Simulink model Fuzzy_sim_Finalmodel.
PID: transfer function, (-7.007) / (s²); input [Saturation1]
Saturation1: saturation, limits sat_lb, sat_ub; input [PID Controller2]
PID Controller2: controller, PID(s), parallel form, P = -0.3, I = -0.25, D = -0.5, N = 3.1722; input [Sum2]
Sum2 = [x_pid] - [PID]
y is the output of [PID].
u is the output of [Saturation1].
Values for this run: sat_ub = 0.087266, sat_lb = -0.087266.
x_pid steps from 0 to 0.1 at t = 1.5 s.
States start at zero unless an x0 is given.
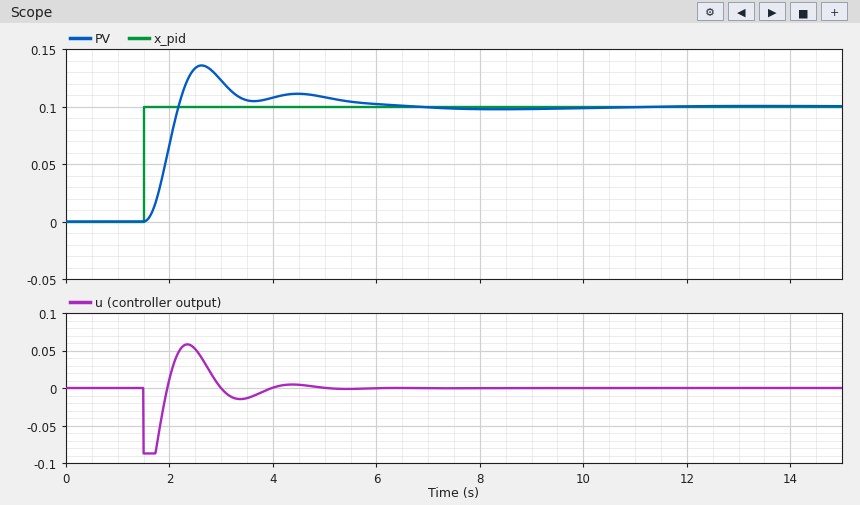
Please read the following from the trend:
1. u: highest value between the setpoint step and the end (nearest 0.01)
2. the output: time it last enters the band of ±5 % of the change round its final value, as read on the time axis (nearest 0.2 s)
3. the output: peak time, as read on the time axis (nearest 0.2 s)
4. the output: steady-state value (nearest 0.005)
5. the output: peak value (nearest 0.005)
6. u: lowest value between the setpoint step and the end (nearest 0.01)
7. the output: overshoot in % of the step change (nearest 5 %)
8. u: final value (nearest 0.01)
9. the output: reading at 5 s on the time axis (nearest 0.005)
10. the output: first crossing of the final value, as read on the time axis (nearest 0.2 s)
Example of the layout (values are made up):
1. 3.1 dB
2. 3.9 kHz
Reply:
1. 0.06
2. 5.4 s
3. 2.6 s
4. 0.100
5. 0.135
6. -0.09
7. 35 %
8. 0.00
9. 0.110
10. 2.2 s
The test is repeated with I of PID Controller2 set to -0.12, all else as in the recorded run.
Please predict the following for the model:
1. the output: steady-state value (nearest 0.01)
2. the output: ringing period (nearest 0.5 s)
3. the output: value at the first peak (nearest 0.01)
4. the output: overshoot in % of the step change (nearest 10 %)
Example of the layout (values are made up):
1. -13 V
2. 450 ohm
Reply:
1. 0.10
2. 2.0 s
3. 0.13
4. 30 %
